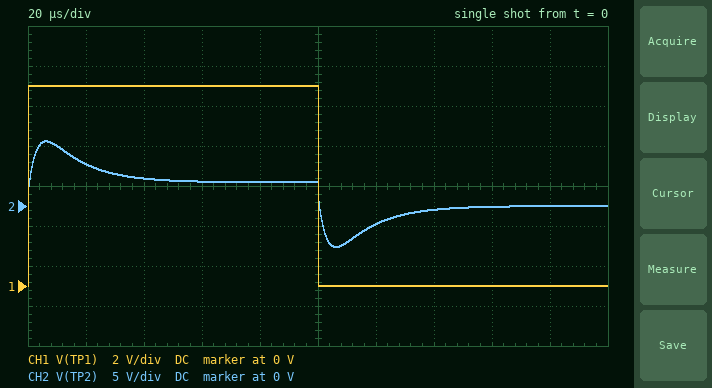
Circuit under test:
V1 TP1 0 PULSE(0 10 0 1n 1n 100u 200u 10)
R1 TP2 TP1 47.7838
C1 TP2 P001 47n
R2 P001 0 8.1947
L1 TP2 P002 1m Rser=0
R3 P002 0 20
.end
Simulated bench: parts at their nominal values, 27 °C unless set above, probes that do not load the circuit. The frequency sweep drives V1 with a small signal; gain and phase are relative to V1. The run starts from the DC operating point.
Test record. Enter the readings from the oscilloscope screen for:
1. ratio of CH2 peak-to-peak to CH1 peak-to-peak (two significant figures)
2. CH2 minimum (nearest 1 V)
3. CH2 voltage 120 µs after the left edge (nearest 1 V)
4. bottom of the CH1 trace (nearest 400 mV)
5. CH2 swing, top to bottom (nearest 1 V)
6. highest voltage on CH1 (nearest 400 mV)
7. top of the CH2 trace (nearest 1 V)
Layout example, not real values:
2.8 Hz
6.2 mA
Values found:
1.3
-5 V
-2 V
0 V
13 V
10.0 V
8 V
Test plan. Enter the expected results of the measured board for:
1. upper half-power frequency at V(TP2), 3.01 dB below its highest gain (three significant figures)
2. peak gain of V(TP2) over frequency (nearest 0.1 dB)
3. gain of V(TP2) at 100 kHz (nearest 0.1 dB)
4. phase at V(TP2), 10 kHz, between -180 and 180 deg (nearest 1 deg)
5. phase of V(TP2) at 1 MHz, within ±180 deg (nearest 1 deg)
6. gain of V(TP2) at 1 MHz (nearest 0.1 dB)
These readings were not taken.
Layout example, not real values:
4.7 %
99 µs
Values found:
74.5 kHz
-0.5 dB
-5.2 dB
24 deg
-19 deg
-16.0 dB
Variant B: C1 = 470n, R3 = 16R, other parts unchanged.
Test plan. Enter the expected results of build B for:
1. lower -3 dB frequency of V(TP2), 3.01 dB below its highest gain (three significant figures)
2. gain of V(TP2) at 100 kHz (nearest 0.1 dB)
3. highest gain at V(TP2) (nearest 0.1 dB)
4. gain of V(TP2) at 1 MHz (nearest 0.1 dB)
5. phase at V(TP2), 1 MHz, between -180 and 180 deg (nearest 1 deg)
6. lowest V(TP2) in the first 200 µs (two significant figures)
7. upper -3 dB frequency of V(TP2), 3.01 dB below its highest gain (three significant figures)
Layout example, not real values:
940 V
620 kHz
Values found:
3.88 kHz
-16.0 dB
-3.5 dB
-16.7 dB
-2 deg
-2.7 V
14.1 kHz
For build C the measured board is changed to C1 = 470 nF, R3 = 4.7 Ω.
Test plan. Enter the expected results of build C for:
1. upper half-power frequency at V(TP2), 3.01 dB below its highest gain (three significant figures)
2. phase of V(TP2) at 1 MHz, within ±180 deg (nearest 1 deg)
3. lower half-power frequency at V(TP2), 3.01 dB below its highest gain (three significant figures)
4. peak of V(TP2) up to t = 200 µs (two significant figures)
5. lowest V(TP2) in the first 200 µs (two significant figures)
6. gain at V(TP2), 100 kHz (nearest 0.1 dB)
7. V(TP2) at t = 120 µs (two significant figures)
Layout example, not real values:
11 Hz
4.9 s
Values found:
12.4 kHz
-2 deg
4.18 kHz
4.9 V
-4.4 V
-16.0 dB
-4.3 V
